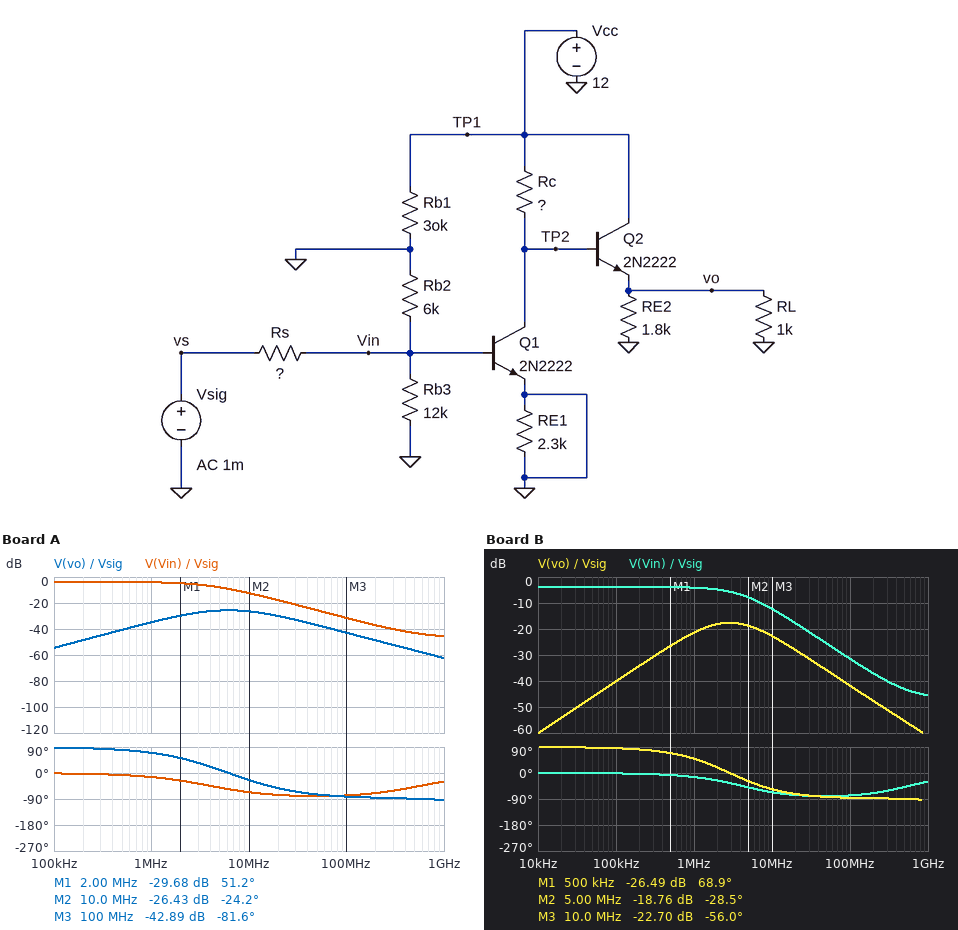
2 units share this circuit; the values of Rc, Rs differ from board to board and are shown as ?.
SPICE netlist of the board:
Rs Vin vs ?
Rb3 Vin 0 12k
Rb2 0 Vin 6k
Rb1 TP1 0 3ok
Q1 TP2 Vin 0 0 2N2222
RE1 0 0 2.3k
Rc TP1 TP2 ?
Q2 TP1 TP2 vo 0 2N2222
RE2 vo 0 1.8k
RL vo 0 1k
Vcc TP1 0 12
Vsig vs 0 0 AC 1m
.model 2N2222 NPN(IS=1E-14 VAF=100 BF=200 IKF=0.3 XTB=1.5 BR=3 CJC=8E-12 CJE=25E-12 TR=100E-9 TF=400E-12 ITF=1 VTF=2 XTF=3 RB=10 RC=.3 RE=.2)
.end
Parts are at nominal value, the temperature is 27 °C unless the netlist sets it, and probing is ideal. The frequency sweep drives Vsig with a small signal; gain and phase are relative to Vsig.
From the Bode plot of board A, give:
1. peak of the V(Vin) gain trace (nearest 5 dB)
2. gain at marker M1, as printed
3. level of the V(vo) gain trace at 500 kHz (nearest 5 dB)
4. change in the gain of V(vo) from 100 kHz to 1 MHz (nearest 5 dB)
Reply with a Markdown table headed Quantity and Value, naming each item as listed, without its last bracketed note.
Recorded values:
| Quantity | Value |
|---|---|
| peak of the V(Vin) gain trace | -5 dB |
| gain at marker M1, as printed | -29.68 dB |
| level of the V(vo) gain trace at 500 kHz | -40 dB |
| change in the gain of V(vo) from 100 kHz to 1 MHz | 20 dB |
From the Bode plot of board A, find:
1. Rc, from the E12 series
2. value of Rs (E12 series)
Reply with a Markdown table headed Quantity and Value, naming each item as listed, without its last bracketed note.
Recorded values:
| Quantity | Value |
|---|---|
| Rc, from the E12 series | 1.5 kΩ |
| value of Rs | 2.2 kΩ |
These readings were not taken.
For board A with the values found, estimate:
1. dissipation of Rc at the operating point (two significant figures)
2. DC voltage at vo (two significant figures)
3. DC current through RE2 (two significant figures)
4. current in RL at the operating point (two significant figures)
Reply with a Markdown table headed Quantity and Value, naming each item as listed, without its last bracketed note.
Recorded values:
| Quantity | Value |
|---|---|
| dissipation of Rc at the operating point | 12 µW |
| DC voltage at vo | 11 V |
| DC current through RE2 | 6.2 mA |
| current in RL at the operating point | 11 mA |
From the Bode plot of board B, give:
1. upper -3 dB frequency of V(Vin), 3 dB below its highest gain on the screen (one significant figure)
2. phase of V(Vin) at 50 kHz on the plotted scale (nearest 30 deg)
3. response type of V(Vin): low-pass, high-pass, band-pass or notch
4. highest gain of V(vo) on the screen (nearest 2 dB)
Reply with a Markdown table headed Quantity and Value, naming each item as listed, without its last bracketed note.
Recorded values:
| Quantity | Value |
|---|---|
| upper -3 dB frequency of V(Vin), 3 dB below its highest gain on the screen | 4 MHz |
| phase of V(Vin) at 50 kHz on the plotted scale | 0 deg |
| response type of V(Vin): low-pass, high-pass, band-pass or notch | low-pass |
| highest gain of V(vo) on the screen | -18 dB |
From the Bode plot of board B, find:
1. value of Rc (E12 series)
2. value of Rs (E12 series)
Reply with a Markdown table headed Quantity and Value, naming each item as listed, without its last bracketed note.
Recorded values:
| Quantity | Value |
|---|---|
| value of Rc | 8.2 kΩ |
| value of Rs | 2.2 kΩ |
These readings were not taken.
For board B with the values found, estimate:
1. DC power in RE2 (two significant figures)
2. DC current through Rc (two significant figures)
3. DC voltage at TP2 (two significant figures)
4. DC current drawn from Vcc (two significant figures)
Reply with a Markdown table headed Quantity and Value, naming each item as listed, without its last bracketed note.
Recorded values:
| Quantity | Value |
|---|---|
| DC power in RE2 | 62 mW |
| DC current through Rc | 86 µA |
| DC voltage at TP2 | 11 V |
| DC current drawn from Vcc | 4.0 A |
